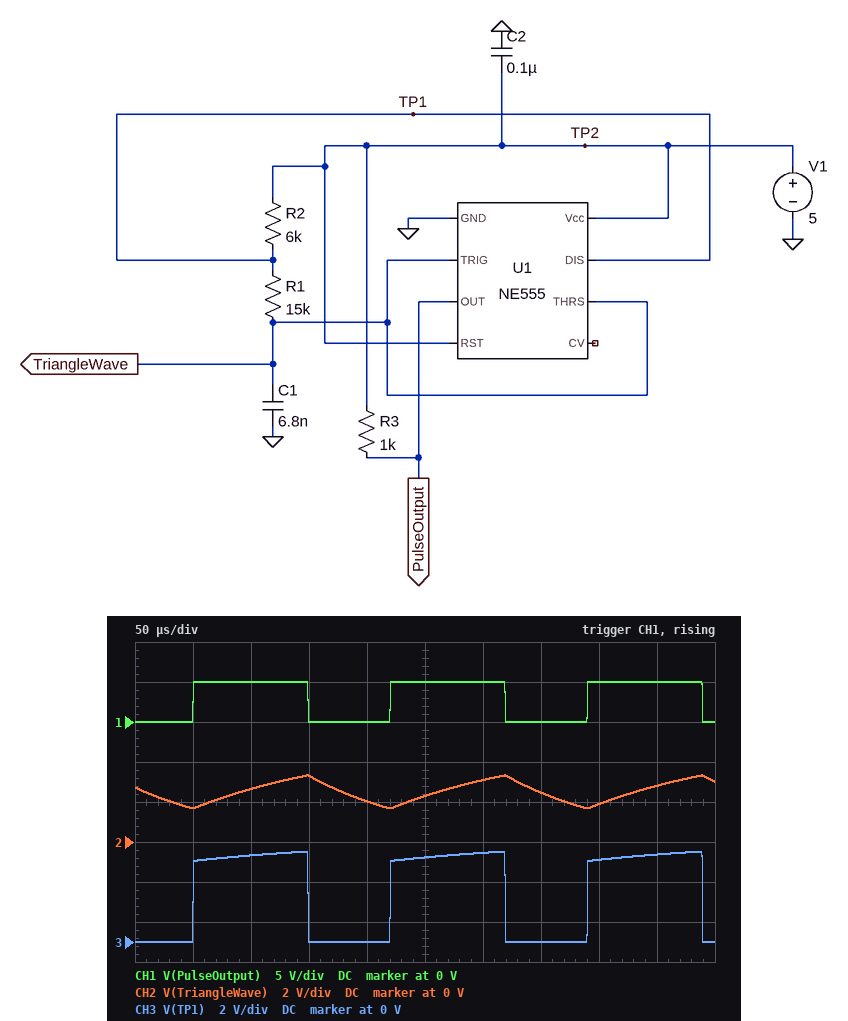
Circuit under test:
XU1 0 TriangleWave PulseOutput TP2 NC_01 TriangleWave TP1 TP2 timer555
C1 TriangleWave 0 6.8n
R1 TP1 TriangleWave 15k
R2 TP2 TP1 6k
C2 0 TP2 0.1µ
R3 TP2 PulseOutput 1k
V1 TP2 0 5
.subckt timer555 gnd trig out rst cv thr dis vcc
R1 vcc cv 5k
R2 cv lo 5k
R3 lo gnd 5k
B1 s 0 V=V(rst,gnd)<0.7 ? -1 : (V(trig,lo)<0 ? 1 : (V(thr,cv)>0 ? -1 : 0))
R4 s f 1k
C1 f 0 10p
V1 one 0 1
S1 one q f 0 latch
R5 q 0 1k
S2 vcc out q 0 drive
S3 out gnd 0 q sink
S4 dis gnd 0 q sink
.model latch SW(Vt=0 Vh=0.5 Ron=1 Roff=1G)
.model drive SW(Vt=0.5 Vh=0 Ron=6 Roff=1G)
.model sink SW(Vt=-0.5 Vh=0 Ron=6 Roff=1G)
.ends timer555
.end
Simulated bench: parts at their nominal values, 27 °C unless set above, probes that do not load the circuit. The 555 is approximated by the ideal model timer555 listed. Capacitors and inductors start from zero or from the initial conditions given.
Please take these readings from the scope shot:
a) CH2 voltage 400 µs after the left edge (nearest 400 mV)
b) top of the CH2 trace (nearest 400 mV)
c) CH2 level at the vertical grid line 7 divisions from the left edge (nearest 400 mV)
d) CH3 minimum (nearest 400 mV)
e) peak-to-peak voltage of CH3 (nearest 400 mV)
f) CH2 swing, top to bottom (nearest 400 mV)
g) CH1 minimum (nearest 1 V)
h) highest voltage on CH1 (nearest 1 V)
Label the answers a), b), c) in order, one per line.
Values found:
a) 2.0 V
b) 3.2 V
c) 2.4 V
d) 0 V
e) 4.4 V
f) 1.6 V
g) 0 V
h) 5 V
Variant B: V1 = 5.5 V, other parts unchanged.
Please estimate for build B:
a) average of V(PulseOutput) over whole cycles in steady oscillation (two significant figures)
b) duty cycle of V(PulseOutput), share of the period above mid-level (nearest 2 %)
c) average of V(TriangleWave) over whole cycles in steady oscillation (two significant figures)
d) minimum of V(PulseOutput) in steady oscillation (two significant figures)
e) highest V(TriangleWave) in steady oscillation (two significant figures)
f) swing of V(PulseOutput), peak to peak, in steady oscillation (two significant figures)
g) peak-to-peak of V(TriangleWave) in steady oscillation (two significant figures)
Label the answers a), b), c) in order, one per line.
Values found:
a) 3.2 V
b) 58 %
c) 2.8 V
d) 33 mV
e) 3.7 V
f) 5.5 V
g) 1.8 V
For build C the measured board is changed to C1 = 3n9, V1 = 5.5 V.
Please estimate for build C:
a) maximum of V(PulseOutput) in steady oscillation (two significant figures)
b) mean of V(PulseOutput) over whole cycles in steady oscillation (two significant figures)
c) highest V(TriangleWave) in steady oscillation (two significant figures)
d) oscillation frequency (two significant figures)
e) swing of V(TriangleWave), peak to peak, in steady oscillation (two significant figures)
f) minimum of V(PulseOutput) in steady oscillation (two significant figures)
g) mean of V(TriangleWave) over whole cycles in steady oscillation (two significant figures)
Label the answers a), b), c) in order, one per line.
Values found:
a) 5.5 V
b) 3.2 V
c) 3.7 V
d) 10 kHz
e) 1.8 V
f) 33 mV
g) 2.8 V
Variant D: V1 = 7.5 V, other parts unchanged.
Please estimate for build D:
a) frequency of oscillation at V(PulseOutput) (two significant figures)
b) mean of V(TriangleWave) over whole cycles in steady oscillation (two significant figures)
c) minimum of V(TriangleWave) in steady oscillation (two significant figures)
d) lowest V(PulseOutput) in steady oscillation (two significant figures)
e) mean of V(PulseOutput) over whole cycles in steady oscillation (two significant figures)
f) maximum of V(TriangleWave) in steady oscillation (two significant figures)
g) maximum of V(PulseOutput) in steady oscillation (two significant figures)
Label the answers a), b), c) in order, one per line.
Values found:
a) 5.9 kHz
b) 3.8 V
c) 2.5 V
d) 45 mV
e) 4.4 V
f) 5.0 V
g) 7.5 V
